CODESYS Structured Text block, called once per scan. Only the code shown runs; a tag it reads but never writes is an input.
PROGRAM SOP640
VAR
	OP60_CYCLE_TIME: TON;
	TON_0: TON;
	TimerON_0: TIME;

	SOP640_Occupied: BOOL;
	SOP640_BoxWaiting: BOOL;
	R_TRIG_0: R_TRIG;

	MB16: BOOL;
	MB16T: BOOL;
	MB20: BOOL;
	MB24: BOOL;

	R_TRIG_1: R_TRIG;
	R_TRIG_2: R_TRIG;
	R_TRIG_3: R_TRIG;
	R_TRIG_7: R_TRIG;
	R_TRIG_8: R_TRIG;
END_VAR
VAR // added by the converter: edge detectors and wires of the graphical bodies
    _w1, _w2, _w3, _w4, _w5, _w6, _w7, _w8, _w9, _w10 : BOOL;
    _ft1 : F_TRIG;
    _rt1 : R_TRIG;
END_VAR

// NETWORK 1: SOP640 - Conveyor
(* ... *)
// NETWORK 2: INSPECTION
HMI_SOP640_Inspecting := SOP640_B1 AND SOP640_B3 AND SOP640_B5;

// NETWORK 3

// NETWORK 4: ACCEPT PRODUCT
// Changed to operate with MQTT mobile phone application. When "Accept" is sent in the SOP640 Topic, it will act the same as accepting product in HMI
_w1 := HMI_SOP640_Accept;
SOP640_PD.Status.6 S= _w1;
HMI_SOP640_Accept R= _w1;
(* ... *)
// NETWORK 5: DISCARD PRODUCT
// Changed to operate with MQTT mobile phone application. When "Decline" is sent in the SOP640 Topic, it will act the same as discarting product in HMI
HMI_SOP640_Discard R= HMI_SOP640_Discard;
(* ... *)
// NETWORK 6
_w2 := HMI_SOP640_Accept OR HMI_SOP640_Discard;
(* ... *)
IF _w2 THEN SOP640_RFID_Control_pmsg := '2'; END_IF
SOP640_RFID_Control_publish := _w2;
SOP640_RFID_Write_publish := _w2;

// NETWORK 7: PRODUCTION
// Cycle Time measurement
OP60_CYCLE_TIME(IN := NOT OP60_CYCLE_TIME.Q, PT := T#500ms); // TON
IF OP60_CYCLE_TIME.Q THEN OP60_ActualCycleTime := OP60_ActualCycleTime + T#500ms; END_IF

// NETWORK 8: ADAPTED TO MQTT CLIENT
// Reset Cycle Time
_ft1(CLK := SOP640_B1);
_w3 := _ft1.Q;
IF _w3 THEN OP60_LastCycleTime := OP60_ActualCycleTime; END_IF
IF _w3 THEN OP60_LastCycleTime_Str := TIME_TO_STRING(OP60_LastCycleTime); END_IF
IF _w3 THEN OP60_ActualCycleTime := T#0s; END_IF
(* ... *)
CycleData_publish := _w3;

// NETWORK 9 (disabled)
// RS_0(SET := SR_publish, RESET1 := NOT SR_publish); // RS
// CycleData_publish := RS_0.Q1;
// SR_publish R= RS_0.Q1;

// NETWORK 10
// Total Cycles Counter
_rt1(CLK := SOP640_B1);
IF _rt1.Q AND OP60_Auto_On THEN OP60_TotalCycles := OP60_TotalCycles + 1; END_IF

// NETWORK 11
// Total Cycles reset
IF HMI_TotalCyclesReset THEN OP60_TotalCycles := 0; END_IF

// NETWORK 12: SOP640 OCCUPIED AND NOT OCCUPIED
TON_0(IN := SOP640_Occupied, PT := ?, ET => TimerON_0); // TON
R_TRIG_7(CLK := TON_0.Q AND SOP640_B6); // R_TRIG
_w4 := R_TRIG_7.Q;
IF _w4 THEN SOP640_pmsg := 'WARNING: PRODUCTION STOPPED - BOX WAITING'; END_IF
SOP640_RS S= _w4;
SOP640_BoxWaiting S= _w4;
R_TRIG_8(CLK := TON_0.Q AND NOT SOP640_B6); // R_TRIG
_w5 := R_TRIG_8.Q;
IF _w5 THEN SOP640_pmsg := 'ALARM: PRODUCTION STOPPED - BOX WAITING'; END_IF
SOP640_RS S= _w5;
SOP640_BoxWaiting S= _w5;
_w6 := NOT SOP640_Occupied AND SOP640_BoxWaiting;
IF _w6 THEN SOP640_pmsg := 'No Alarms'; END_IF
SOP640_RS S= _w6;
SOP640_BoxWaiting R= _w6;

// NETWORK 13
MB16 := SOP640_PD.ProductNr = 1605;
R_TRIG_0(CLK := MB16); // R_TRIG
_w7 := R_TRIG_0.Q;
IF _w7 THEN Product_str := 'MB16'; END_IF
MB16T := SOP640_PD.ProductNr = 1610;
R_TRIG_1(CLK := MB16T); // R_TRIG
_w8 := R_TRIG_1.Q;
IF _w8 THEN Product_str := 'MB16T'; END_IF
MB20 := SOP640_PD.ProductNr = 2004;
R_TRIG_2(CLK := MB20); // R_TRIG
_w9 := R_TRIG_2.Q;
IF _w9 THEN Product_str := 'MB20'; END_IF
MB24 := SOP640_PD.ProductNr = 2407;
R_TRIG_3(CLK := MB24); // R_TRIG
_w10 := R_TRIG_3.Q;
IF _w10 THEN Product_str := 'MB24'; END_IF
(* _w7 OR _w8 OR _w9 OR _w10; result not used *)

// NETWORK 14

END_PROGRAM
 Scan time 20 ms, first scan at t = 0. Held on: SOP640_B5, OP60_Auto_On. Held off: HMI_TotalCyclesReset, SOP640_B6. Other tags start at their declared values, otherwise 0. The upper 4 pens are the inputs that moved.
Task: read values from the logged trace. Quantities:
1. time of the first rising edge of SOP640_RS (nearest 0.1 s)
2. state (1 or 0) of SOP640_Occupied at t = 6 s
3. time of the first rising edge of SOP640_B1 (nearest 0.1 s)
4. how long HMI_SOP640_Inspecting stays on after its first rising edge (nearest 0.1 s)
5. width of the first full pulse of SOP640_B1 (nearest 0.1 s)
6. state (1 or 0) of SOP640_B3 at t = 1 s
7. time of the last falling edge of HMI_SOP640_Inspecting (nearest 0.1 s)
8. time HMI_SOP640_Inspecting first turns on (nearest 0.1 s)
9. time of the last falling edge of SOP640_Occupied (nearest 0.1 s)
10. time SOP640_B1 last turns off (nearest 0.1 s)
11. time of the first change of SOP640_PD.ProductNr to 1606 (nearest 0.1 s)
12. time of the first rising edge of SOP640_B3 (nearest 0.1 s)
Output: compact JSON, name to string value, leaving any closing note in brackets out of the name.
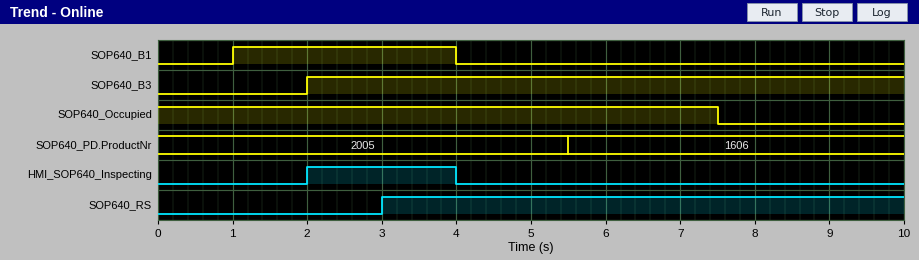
{"time of the first rising edge of SOP640_RS": "3.0 s", "state (1 or 0) of SOP640_Occupied at t = 6 s": "1", "time of the first rising edge of SOP640_B1": "1.0 s", "how long HMI_SOP640_Inspecting stays on after its first rising edge": "2.0 s", "width of the first full pulse of SOP640_B1": "3.0 s", "state (1 or 0) of SOP640_B3 at t = 1 s": "0", "time of the last falling edge of HMI_SOP640_Inspecting": "4.0 s", "time HMI_SOP640_Inspecting first turns on": "2.0 s", "time of the last falling edge of SOP640_Occupied": "7.5 s", "time SOP640_B1 last turns off": "4.0 s", "time of the first change of SOP640_PD.ProductNr to 1606": "5.5 s", "time of the first rising edge of SOP640_B3": "2.0 s"}
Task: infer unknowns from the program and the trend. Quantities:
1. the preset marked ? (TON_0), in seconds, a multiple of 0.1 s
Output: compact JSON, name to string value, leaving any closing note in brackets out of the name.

{"the preset marked ? (TON_0), in seconds, a multiple of 0.1 s": "3.0 s"}
